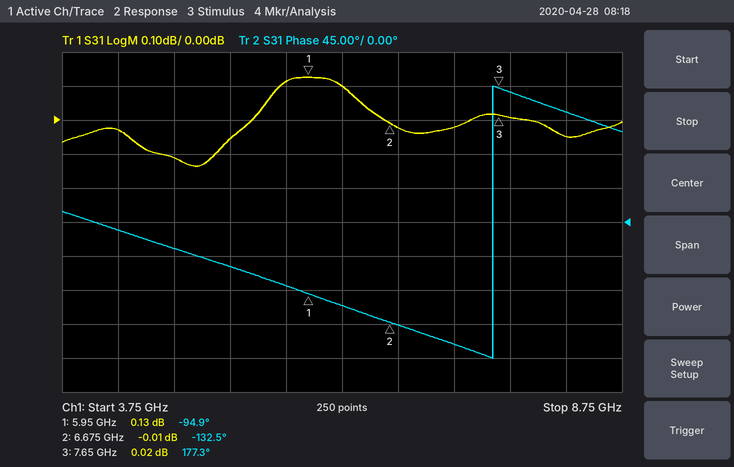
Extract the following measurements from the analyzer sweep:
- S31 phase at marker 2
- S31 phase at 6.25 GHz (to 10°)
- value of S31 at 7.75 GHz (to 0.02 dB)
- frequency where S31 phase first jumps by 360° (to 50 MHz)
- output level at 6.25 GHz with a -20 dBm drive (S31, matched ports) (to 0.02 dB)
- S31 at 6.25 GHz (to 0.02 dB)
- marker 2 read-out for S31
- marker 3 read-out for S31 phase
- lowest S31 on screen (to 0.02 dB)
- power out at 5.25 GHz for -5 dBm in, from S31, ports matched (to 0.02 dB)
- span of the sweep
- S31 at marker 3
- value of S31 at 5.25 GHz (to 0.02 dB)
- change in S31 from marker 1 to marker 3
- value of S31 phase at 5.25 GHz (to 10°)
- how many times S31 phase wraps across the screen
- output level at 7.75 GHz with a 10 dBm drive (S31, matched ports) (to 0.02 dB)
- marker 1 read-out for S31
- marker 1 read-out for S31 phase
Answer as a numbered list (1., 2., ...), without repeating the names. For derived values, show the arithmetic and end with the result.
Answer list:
1. -132.5°
2. -110°
3. 0.00 dB
4. 7.60 GHz
5. -20 dBm + (0.10 dB) = -19.90 dBm
6. 0.10 dB
7. -0.01 dB
8. 177.3°
9. -0.14 dB
10. -5 dBm + (-0.06 dB) = -5.06 dBm
11. 5 GHz
12. 0.02 dB
13. -0.06 dB
14. 0.02 − (0.13) = -0.11 dB
15. -60°
16. 1
17. 10 dBm + (0.00 dB) = 10.00 dBm
18. 0.13 dB
19. -94.9°
